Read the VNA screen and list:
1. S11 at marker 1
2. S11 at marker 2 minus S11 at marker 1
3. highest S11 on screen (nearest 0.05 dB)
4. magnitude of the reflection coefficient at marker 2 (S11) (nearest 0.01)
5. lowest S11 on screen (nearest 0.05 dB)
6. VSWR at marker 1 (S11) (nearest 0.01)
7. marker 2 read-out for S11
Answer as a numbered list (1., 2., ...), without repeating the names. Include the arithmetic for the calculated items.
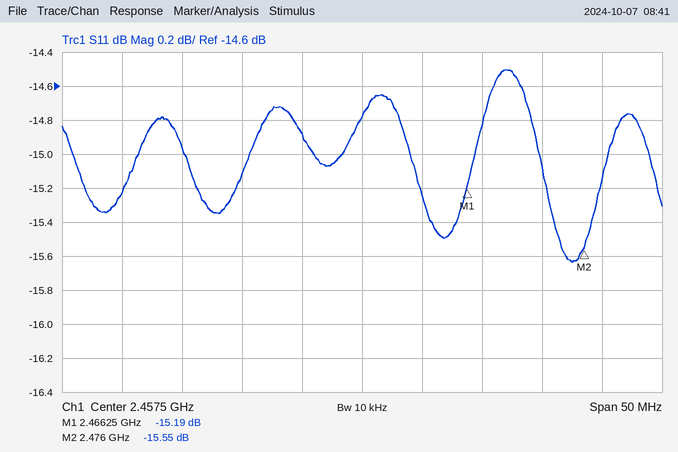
1. -15.19 dB
2. -15.55 − (-15.19) = -0.36 dB
3. -14.50 dB
4. 10^(-15.55/20) ≈ 0.17
5. -15.65 dB
6. (1 + 0.1740)/(1 − 0.1740) ≈ 1.42
7. -15.55 dB
